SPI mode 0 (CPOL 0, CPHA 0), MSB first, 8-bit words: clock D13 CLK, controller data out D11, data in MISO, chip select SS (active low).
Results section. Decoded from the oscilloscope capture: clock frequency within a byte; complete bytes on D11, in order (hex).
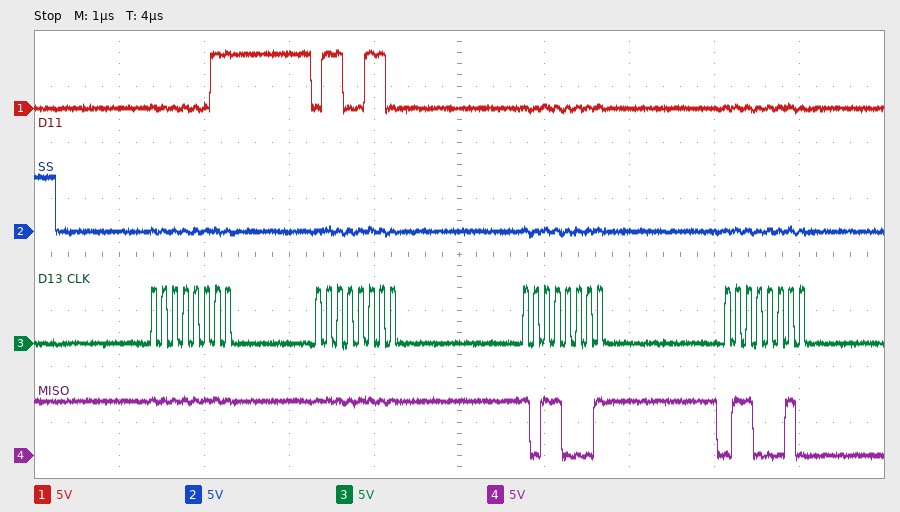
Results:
8 MHz
03 66 00 00
